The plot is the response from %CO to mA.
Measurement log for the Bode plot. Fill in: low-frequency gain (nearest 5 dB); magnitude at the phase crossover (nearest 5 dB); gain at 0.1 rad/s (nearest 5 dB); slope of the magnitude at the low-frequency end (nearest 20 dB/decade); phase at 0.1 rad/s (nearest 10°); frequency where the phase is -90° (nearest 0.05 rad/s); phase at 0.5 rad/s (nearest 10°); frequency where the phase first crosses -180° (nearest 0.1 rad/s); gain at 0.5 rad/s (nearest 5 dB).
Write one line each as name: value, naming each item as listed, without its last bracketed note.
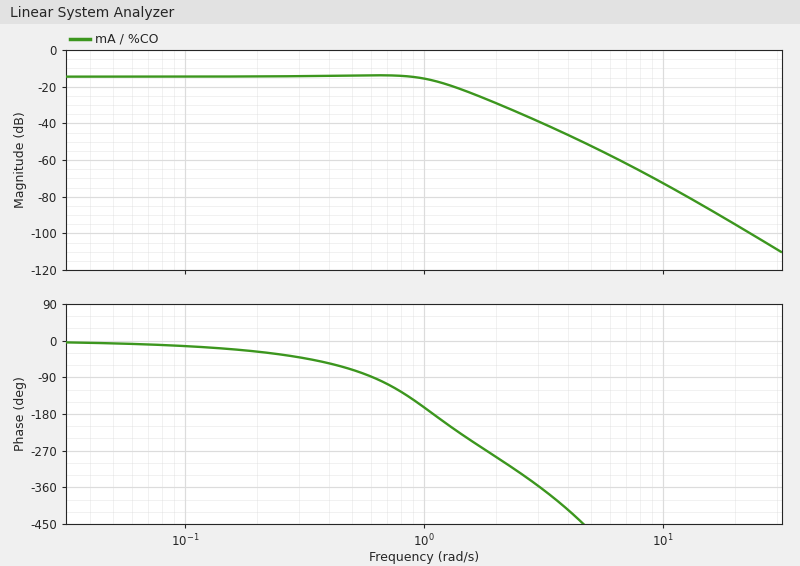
low-frequency gain: -15 dB
magnitude at the phase crossover: -15 dB
gain at 0.1 rad/s: -15 dB
slope of the magnitude at the low-frequency end: 0 dB/decade
phase at 0.1 rad/s: -10°
frequency where the phase is -90°: 0.60 rad/s
phase at 0.5 rad/s: -70°
frequency where the phase first crosses -180°: 1.1 rad/s
gain at 0.5 rad/s: -15 dB
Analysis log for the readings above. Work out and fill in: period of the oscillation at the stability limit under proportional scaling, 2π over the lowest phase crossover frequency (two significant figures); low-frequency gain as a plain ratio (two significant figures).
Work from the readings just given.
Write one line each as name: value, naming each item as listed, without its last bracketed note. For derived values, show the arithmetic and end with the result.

period of the oscillation at the stability limit under proportional scaling, 2π over the lowest phase crossover frequency: 2π / 1.1 = 5.7 s
low-frequency gain as a plain ratio: 10^(-15 / 20) = 0.18
